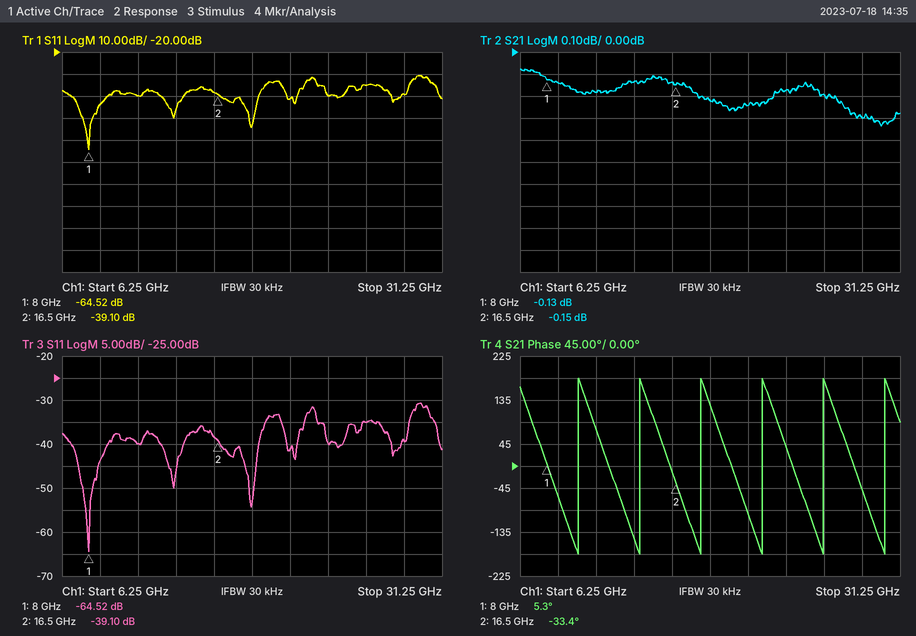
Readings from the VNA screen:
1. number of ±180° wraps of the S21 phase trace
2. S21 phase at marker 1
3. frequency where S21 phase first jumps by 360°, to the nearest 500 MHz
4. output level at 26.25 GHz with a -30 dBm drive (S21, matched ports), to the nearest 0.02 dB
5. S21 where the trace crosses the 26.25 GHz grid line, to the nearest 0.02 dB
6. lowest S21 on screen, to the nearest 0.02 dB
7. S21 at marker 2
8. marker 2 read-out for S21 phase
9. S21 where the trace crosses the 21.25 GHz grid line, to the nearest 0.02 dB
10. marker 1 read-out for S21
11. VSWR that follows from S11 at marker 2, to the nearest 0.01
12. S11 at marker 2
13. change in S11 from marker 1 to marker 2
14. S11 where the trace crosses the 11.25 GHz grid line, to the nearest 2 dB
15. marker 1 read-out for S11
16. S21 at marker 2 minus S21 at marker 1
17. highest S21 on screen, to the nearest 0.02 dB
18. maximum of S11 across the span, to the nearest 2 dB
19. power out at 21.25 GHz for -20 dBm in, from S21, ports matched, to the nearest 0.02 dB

6
5.3°
10.0 GHz
-30.20 dBm
-0.20 dB
-0.34 dB
-0.15 dB
-33.4°
-0.24 dB
-0.13 dB
1.02
-39.10 dB
25.42 dB
-40 dB
-64.52 dB
-0.02 dB
-0.08 dB
-30 dB
-20.24 dBm
